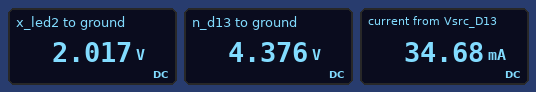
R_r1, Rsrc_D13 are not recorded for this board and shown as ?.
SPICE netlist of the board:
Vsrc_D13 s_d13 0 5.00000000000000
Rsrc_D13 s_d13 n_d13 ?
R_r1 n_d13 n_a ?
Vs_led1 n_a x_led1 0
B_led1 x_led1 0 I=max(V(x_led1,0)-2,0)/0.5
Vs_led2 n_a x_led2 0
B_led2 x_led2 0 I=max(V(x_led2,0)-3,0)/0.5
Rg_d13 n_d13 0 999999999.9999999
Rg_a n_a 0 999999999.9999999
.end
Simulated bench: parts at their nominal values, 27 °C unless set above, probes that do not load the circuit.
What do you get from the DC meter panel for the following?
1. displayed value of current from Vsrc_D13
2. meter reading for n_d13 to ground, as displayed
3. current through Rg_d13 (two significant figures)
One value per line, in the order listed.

34.68 mA
4.376 V
4.4 nA
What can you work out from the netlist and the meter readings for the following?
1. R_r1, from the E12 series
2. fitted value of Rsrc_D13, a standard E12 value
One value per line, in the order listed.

68 Ω
18 Ω
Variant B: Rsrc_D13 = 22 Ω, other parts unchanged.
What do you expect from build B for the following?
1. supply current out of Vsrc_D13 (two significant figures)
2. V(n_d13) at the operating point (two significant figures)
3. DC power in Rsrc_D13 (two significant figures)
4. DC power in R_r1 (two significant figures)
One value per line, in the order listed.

33 mA
4.3 V
24 mW
75 mW
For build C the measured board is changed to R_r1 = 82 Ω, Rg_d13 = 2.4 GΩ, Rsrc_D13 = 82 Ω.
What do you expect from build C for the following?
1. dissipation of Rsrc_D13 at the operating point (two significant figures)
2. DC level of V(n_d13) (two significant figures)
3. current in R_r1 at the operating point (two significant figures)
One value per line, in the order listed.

27 mW
3.5 V
18 mA
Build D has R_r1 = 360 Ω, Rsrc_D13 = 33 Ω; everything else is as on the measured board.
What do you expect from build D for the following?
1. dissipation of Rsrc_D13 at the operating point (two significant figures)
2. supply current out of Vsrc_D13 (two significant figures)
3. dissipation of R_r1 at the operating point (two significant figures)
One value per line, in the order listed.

1.9 mW
7.6 mA
21 mW
